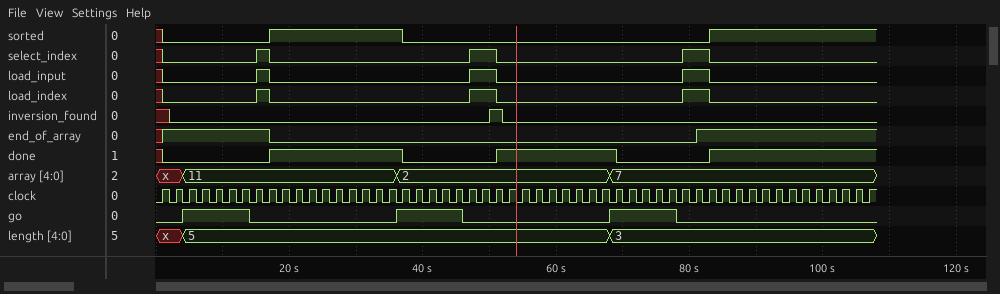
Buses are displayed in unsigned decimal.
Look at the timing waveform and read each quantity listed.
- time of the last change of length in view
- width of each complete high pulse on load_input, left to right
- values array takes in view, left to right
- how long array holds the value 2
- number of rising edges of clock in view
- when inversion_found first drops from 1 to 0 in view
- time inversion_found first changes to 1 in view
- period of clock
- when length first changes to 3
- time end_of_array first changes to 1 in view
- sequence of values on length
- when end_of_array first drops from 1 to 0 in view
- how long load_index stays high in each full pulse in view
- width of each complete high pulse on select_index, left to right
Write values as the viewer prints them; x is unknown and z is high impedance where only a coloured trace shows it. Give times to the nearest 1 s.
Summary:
68 s
2 s, 4 s, 4 s
x, 11, 2, 7
32 s
54
52 s
50 s
2 s
68 s
1 s
x, 5, 3
17 s
2 s, 4 s, 4 s
2 s, 4 s, 4 s
